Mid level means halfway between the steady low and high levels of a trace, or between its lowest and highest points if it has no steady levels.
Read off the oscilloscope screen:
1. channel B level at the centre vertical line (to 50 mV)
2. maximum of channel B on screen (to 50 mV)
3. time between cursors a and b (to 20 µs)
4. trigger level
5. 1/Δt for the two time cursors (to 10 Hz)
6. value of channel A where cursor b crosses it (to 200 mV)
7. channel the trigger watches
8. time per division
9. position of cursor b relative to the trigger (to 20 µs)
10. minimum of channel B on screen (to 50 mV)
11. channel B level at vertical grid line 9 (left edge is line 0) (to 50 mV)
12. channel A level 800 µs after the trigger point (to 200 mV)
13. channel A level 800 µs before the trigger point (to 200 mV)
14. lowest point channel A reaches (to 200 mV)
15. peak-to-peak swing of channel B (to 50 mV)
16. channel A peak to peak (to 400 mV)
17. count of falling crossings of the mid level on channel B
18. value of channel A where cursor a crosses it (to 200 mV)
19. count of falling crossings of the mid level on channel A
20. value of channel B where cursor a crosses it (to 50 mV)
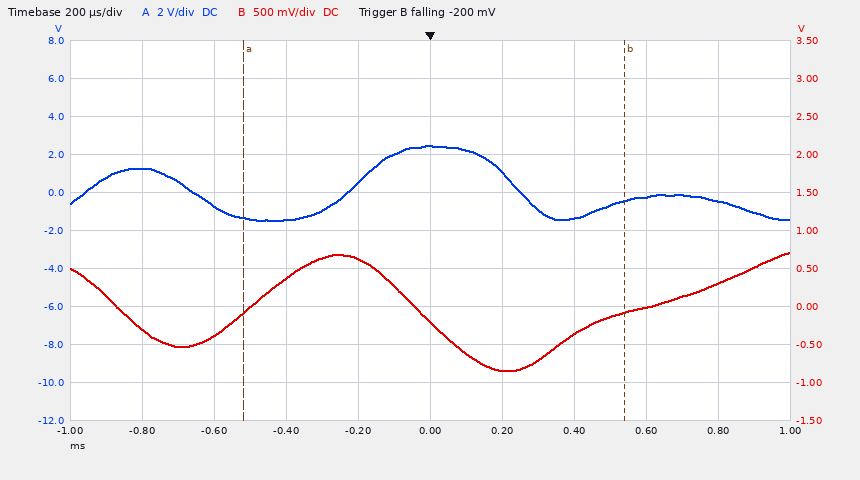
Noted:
-200 mV
700 mV
1.06 ms
-200 mV
940 Hz
-400 mV
channel B
200 µs
+540 µs
-850 mV
300 mV
-400 mV
1.2 V
-1.4 V
1.55 V
4.0 V
2
-1.4 V
2
-100 mV
